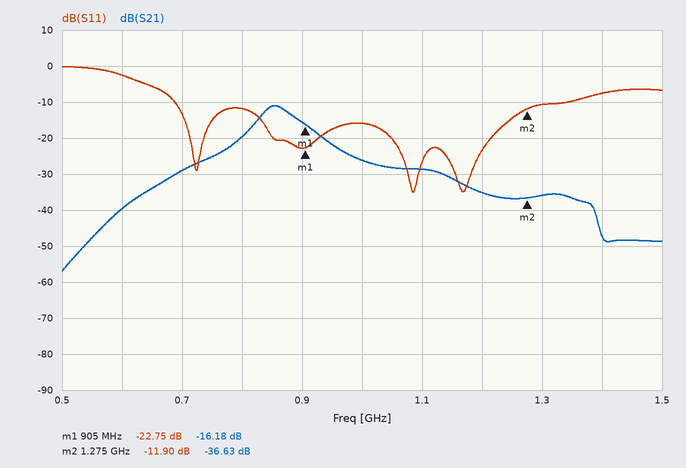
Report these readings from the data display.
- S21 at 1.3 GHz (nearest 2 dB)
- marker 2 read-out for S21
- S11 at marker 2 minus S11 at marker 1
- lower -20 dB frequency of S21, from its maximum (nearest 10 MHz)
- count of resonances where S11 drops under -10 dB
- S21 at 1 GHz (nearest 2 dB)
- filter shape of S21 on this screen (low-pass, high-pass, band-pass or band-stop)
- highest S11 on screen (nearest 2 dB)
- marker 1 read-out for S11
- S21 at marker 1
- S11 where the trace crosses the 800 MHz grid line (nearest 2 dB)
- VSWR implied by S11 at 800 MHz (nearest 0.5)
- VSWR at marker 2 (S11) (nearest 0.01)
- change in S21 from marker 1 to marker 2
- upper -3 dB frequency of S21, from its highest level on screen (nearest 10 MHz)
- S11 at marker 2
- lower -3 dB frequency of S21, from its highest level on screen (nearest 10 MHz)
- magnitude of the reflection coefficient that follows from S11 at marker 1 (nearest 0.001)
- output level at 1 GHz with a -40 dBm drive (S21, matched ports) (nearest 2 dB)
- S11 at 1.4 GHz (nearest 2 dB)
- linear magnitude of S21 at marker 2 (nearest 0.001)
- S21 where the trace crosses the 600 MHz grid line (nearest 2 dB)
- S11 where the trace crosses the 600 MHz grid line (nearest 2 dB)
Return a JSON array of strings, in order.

["-36 dB", "-36.63 dB", "10.85 dB", "680 MHz", "4", "-26 dB", "band-pass", "0 dB", "-22.75 dB", "-16.18 dB", "-12 dB", "1.5", "1.68", "-20.45 dB", "890 MHz", "-11.90 dB", "830 MHz", "0.073", "-66 dBm", "-8 dB", "0.015", "-40 dB", "-2 dB"]
